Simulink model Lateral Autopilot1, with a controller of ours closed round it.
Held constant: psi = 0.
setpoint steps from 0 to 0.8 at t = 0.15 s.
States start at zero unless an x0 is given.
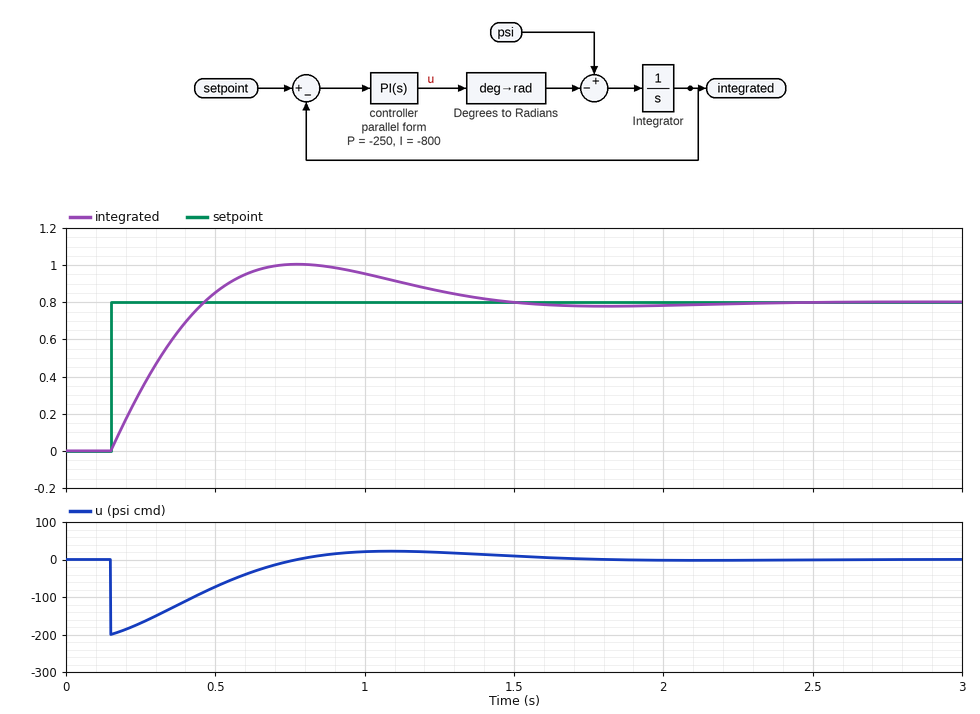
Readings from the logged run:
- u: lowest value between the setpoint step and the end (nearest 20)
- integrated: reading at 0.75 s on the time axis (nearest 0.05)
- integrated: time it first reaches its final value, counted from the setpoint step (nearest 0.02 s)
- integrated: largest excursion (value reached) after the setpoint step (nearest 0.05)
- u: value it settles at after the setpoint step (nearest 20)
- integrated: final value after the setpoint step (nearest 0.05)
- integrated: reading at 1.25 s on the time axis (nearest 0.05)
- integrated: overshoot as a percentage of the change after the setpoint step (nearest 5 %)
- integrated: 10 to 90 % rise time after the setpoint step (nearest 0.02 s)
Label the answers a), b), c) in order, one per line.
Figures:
a) -200
b) 1.00
c) 0.32 s
d) 1.00
e) 0
f) 0.80
g) 0.85
h) 25 %
i) 0.24 s
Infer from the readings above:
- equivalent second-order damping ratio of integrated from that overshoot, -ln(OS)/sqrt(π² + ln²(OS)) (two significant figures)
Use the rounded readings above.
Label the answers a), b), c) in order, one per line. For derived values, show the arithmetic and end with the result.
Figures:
a) ln(0.25) = -1.386; 1.386 / sqrt(9.870 + 1.922) = 0.40
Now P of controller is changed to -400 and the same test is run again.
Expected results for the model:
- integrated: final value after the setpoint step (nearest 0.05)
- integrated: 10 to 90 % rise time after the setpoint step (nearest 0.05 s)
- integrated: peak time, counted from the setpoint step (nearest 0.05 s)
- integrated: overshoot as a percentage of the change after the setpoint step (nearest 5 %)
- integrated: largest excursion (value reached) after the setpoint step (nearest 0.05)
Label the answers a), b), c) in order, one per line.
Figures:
a) 0.80
b) 0.20 s
c) 0.55 s
d) 15 %
e) 0.90
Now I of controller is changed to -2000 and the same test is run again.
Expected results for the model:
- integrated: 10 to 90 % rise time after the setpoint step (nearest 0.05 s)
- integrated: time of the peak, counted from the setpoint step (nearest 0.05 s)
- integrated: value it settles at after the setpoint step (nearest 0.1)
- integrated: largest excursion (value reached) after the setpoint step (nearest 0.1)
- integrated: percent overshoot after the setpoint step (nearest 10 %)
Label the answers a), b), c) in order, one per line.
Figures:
a) 0.15 s
b) 0.45 s
c) 0.8
d) 1.1
e) 40 %
